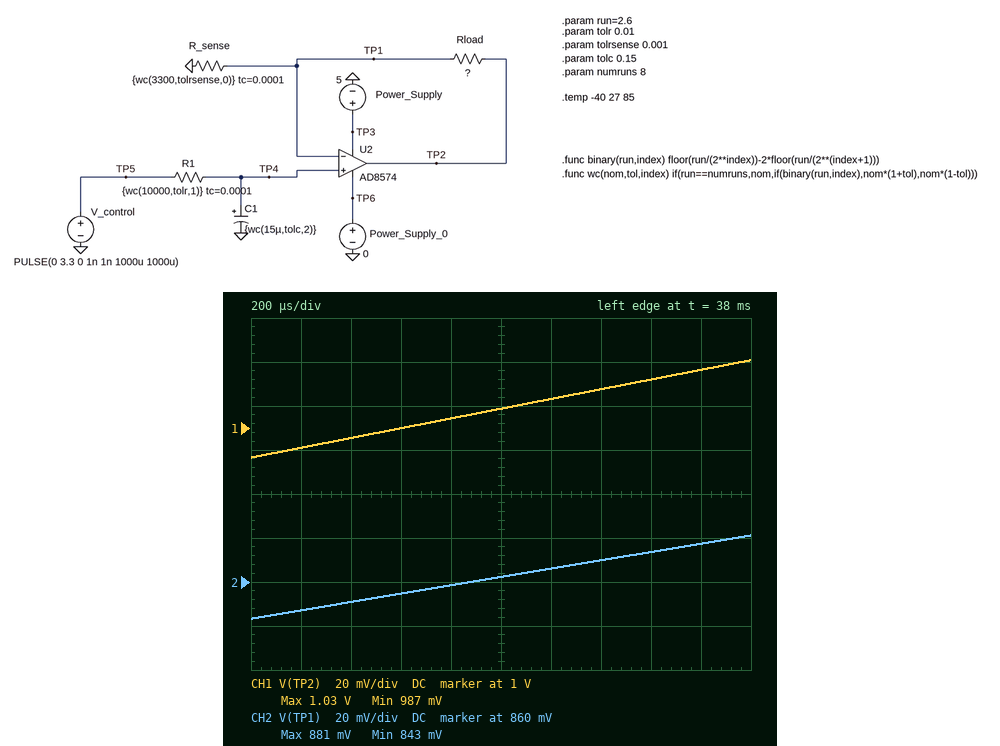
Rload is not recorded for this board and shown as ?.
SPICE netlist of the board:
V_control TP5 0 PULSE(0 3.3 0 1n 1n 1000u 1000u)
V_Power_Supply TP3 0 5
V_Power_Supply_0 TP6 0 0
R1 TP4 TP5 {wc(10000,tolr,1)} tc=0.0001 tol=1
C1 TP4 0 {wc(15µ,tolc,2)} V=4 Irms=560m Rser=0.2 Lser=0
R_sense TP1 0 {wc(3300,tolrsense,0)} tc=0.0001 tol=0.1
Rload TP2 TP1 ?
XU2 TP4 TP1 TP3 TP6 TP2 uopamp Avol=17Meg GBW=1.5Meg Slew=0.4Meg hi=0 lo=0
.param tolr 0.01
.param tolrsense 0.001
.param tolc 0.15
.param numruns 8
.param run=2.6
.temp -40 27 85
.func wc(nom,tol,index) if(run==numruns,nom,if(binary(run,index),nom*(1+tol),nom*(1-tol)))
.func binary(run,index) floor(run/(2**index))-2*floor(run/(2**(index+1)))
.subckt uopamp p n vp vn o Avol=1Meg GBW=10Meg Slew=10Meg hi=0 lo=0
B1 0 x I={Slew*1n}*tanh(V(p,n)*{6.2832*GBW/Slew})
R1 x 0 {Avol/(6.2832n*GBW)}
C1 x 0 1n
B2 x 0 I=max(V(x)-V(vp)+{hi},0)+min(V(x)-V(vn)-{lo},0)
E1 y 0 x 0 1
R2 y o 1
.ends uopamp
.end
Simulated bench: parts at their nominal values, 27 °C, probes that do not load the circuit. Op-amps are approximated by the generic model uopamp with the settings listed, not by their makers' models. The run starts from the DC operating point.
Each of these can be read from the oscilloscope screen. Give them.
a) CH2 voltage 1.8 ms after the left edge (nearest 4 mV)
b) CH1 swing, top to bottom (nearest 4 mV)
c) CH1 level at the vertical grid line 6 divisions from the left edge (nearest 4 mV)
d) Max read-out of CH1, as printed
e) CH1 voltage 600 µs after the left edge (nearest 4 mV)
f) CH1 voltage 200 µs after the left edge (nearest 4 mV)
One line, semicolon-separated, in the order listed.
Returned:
876 mV; 44 mV; 1.012 V; 1.03 V; 1.000 V; 992 mV
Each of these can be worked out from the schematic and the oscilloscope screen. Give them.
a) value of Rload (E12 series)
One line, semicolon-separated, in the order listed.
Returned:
560 Ω
